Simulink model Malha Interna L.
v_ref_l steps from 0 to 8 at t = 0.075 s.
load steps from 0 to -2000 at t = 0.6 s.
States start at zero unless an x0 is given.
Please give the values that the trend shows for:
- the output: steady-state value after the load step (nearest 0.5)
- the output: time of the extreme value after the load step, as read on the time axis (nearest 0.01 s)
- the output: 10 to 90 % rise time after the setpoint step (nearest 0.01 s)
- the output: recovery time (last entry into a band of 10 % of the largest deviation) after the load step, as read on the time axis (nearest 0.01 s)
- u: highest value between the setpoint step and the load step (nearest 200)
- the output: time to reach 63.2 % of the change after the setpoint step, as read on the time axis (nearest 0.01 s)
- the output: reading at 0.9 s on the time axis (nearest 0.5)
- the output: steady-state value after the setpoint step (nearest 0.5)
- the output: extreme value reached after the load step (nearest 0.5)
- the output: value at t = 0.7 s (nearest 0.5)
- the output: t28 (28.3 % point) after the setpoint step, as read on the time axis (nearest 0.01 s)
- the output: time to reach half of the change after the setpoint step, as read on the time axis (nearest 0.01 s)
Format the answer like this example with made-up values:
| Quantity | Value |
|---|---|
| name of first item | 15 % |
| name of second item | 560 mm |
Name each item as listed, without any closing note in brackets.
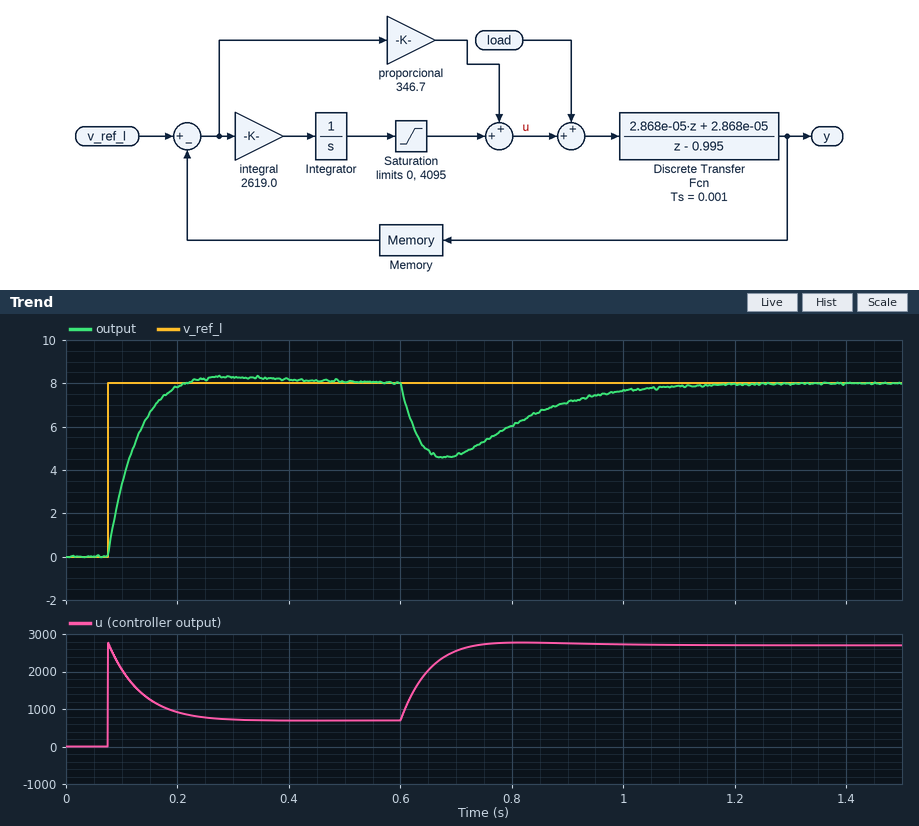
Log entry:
| Quantity | Value |
|---|---|
| the output: steady-state value after the load step | 8.0 |
| the output: time of the extreme value after the load step, as read on the time axis | 0.68 s |
| the output: 10 to 90 % rise time after the setpoint step | 0.09 s |
| the output: recovery time (last entry into a band of 10 % of the largest deviation) after the load step, as read on the time axis | 1.00 s |
| u: highest value between the setpoint step and the load step | 2800 |
| the output: time to reach 63.2 % of the change after the setpoint step, as read on the time axis | 0.12 s |
| the output: reading at 0.9 s on the time axis | 7.0 |
| the output: steady-state value after the setpoint step | 8.0 |
| the output: extreme value reached after the load step | 4.5 |
| the output: value at t = 0.7 s | 4.5 |
| the output: t28 (28.3 % point) after the setpoint step, as read on the time axis | 0.09 s |
| the output: time to reach half of the change after the setpoint step, as read on the time axis | 0.11 s |
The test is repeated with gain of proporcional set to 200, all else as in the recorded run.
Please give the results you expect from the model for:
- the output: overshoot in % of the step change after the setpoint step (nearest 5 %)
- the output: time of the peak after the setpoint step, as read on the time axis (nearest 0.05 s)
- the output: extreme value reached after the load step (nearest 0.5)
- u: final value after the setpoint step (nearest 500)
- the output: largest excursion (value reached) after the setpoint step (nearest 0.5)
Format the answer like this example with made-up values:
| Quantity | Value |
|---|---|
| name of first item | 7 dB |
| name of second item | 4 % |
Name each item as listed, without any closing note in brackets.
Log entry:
| Quantity | Value |
|---|---|
| the output: overshoot in % of the step change after the setpoint step | 10 % |
| the output: time of the peak after the setpoint step, as read on the time axis | 0.30 s |
| the output: extreme value reached after the load step | 3.5 |
| u: final value after the setpoint step | 500 |
| the output: largest excursion (value reached) after the setpoint step | 9.0 |
